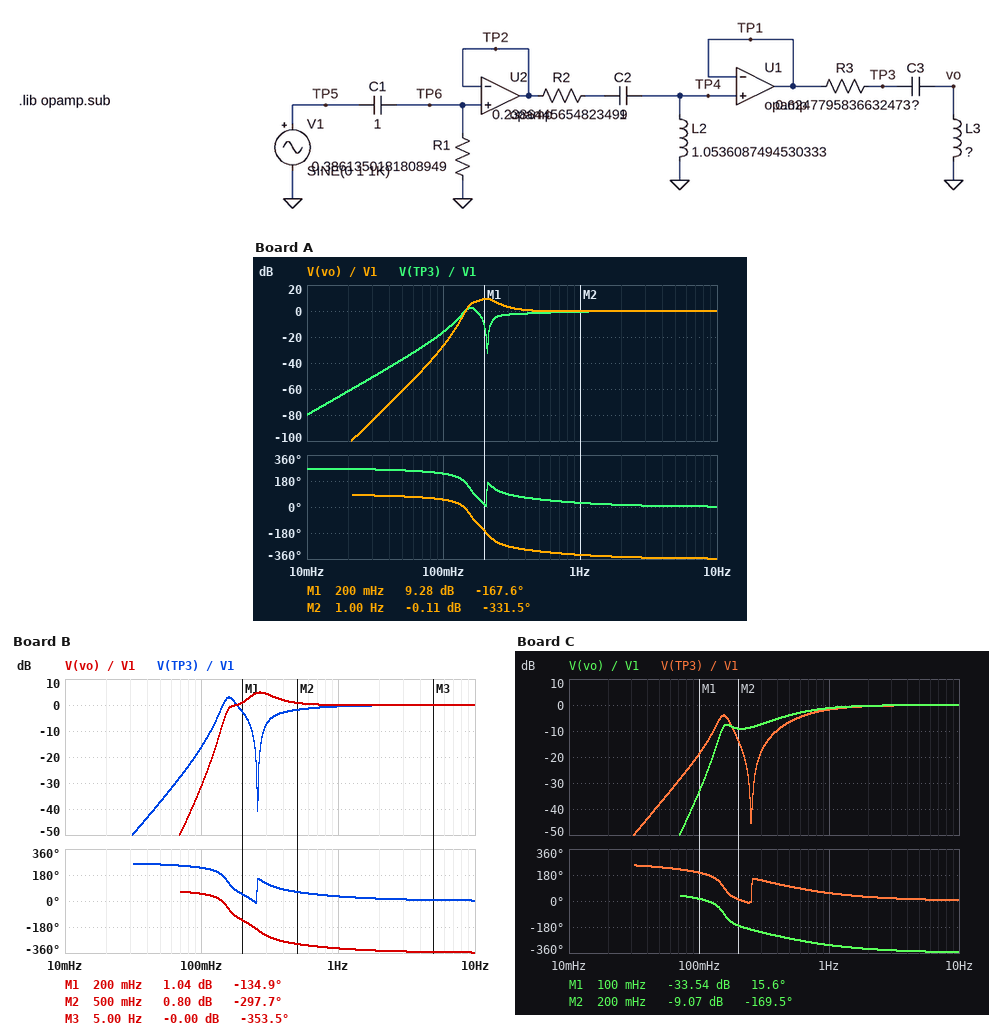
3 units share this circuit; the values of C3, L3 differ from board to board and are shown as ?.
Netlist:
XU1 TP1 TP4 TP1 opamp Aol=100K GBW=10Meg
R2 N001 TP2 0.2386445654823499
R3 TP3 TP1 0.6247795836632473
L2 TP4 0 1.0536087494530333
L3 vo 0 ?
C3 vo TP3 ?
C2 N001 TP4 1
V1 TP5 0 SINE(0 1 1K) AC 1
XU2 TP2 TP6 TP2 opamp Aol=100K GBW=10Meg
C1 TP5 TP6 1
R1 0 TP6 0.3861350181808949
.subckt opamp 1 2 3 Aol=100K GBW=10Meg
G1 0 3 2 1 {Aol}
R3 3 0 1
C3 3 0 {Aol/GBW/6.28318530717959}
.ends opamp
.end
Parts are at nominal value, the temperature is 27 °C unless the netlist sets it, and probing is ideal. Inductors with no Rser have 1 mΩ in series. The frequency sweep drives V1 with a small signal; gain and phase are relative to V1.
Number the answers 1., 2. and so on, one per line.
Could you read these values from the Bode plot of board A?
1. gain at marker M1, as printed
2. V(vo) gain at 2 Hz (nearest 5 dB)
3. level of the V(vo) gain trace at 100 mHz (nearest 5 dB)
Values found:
1. 9.28 dB
2. 0 dB
3. -25 dB
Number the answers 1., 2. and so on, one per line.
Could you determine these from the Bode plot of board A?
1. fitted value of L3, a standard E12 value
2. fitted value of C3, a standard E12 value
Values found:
1. 1.5 H
2. 390 mF
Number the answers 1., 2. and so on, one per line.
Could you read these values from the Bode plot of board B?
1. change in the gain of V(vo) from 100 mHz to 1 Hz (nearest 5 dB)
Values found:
1. 30 dB
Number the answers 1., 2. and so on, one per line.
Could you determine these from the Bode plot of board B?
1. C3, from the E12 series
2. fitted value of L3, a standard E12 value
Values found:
1. 470 mF
2. 820 mH
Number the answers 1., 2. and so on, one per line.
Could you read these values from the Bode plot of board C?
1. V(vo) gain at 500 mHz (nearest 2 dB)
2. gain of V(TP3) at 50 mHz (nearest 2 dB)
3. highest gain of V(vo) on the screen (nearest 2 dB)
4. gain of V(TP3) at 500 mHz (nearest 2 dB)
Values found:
1. -4 dB
2. -38 dB
3. 0 dB
4. -6 dB
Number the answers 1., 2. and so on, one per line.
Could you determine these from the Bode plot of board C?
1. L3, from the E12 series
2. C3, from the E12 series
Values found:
1. 180 mH
2. 2.2 F
